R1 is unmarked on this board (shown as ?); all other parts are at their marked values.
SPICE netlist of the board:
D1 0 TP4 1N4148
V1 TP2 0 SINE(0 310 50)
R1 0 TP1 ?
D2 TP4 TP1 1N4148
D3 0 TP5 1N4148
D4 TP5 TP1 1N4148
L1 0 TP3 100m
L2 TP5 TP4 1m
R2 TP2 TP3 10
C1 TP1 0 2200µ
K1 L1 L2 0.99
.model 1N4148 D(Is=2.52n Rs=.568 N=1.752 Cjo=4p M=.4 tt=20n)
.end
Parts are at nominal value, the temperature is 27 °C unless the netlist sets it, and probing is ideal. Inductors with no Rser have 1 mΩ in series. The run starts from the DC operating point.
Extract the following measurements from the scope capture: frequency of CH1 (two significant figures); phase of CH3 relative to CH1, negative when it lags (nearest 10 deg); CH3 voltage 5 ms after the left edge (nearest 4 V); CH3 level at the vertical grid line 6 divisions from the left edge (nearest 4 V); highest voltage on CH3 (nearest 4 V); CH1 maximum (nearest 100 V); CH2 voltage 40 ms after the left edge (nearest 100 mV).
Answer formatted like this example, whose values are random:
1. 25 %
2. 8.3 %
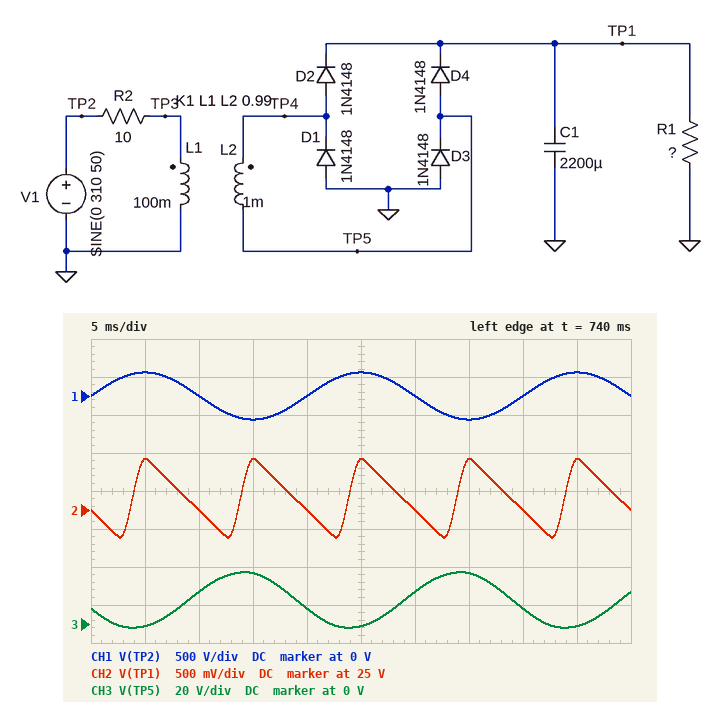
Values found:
1. 50 Hz
2. -160 deg
3. 0 V
4. 16 V
5. 28 V
6. 300 V
7. 25.0 V
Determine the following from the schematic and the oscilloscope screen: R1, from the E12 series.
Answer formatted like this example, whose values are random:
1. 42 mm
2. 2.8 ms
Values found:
1. 82 Ω
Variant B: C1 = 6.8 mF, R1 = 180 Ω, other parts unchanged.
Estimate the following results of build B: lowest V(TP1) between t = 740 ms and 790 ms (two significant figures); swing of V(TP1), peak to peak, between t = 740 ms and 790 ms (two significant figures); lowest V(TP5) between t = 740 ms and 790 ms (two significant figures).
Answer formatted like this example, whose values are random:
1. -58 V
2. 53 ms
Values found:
1. 26 V
2. 170 mV
3. -1.5 V
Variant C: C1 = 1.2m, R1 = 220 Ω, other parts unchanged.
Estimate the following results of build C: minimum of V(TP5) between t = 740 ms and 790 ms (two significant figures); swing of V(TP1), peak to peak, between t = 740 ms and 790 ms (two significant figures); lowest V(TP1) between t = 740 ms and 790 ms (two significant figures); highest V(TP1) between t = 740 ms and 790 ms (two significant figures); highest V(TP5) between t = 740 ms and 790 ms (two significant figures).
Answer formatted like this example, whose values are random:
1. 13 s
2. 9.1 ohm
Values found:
1. -1.4 V
2. 800 mV
3. 26 V
4. 27 V
5. 28 V
